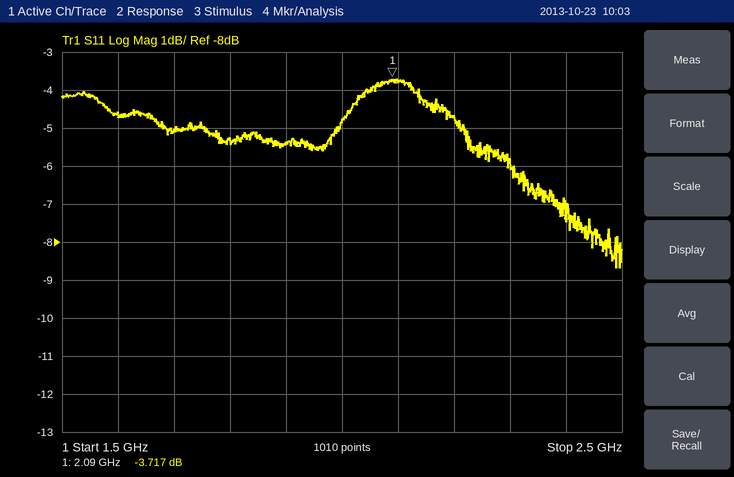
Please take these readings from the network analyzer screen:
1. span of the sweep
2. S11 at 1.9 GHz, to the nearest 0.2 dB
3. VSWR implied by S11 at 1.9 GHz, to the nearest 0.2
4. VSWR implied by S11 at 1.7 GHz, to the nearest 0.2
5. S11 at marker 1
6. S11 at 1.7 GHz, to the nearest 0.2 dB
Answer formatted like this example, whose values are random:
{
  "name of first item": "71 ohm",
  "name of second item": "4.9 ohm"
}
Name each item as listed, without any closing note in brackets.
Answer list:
{
  "span of the sweep": "1 GHz",
  "S11 at 1.9 GHz, to the nearest 0.2 dB": "-5.4 dB",
  "VSWR implied by S11 at 1.9 GHz, to the nearest 0.2": "3.4",
  "VSWR implied by S11 at 1.7 GHz, to the nearest 0.2": "3.6",
  "S11 at marker 1": "-3.717 dB",
  "S11 at 1.7 GHz, to the nearest 0.2 dB": "-5.0 dB"
}
